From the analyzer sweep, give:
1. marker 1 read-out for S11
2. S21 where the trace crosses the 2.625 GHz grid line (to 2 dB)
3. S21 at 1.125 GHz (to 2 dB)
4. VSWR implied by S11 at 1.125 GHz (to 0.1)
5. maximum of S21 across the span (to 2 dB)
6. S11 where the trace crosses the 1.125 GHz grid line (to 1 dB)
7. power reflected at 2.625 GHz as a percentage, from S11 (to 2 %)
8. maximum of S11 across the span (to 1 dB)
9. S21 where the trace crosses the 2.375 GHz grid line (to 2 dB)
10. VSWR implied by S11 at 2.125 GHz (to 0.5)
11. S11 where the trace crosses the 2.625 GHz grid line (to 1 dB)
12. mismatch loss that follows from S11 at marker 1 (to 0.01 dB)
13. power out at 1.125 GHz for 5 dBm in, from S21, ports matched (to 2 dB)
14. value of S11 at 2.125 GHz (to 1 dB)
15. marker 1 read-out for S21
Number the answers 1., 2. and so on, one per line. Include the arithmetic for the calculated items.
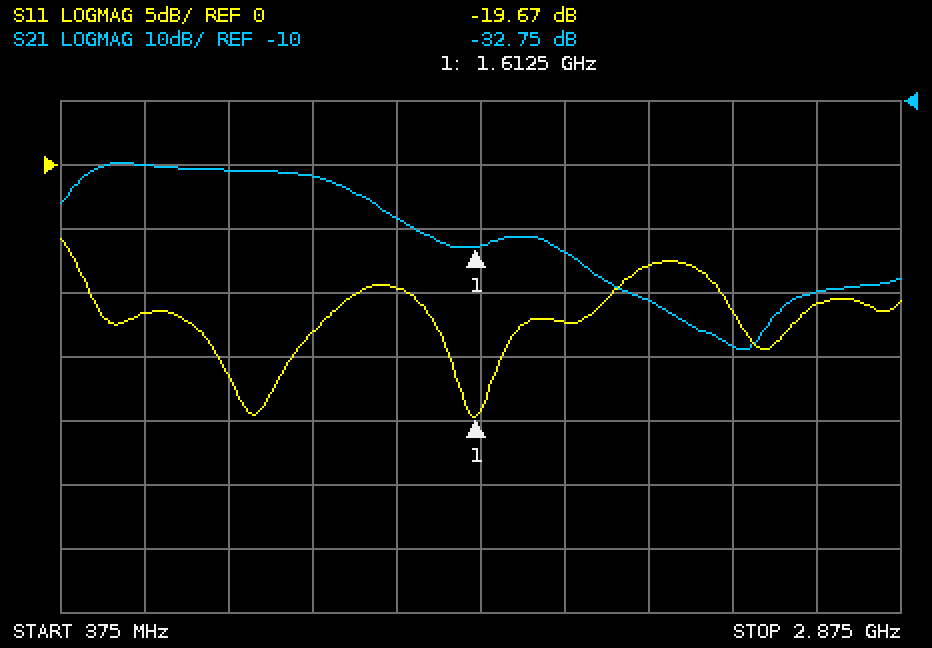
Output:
1. -19.67 dB
2. -40 dB
3. -22 dB
4. |Γ| = 10^(-13/20) = 0.2239; VSWR = (1 + 0.2239)/(1 − 0.2239) ≈ 1.6
5. -20 dB
6. -13 dB
7. 10^(-11/10) ≈ 8 %
8. -6 dB
9. -48 dB
10. |Γ| = 10^(-8/20) = 0.3981; VSWR = (1 + 0.3981)/(1 − 0.3981) ≈ 2.32, so 2.5 to the nearest 0.5
11. -11 dB
12. −10 log10(1 − 10^(-19.67/10)) ≈ 0.05 dB
13. 5 dBm + (-22 dB) = -16 dBm
14. -8 dB
15. -32.75 dB
